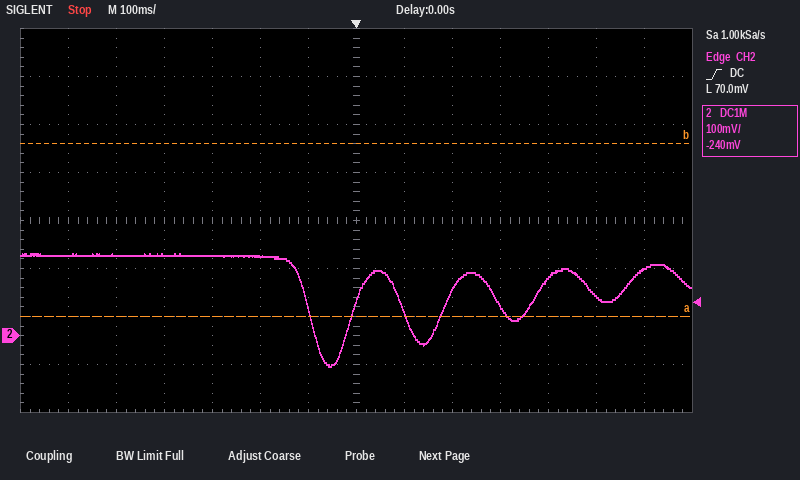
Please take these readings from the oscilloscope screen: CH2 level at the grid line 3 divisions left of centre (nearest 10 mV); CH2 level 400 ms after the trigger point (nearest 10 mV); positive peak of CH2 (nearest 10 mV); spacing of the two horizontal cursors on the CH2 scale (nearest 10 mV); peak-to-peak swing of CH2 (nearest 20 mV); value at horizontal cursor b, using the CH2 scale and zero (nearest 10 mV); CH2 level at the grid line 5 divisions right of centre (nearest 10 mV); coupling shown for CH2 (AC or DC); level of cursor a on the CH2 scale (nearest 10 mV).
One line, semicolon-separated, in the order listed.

170 mV; 120 mV; 170 mV; 360 mV; 240 mV; 400 mV; 80 mV; DC; 40 mV
